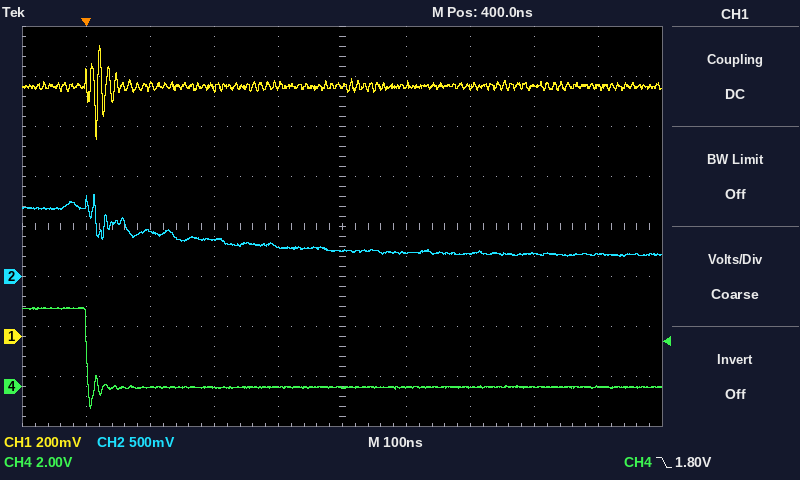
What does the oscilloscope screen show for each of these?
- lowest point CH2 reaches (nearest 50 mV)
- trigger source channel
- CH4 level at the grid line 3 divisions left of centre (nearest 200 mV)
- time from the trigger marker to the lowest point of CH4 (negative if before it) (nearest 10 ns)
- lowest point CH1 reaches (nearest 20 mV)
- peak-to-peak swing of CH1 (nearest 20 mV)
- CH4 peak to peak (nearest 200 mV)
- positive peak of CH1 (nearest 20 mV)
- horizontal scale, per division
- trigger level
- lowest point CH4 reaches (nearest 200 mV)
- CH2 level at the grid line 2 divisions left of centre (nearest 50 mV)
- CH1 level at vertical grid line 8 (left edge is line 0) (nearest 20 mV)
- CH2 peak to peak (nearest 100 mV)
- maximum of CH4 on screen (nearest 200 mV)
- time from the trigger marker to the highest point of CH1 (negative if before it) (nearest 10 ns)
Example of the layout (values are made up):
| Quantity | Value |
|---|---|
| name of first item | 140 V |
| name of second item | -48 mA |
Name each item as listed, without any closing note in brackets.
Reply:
| Quantity | Value |
|---|---|
| lowest point CH2 reaches | 200 mV |
| trigger source channel | CH4 |
| CH4 level at the grid line 3 divisions left of centre | 0.0 V |
| time from the trigger marker to the lowest point of CH4 (negative if before it) | +10 ns |
| lowest point CH1 reaches | 780 mV |
| peak-to-peak swing of CH1 | 380 mV |
| CH4 peak to peak | 4.0 V |
| positive peak of CH1 | 1.16 V |
| horizontal scale, per division | 100 ns |
| trigger level | 1.80 V |
| lowest point CH4 reaches | -800 mV |
| CH2 level at the grid line 2 divisions left of centre | 350 mV |
| CH1 level at vertical grid line 8 (left edge is line 0) | 1.00 V |
| CH2 peak to peak | 600 mV |
| maximum of CH4 on screen | 3.2 V |
| time from the trigger marker to the highest point of CH1 (negative if before it) | +20 ns |
